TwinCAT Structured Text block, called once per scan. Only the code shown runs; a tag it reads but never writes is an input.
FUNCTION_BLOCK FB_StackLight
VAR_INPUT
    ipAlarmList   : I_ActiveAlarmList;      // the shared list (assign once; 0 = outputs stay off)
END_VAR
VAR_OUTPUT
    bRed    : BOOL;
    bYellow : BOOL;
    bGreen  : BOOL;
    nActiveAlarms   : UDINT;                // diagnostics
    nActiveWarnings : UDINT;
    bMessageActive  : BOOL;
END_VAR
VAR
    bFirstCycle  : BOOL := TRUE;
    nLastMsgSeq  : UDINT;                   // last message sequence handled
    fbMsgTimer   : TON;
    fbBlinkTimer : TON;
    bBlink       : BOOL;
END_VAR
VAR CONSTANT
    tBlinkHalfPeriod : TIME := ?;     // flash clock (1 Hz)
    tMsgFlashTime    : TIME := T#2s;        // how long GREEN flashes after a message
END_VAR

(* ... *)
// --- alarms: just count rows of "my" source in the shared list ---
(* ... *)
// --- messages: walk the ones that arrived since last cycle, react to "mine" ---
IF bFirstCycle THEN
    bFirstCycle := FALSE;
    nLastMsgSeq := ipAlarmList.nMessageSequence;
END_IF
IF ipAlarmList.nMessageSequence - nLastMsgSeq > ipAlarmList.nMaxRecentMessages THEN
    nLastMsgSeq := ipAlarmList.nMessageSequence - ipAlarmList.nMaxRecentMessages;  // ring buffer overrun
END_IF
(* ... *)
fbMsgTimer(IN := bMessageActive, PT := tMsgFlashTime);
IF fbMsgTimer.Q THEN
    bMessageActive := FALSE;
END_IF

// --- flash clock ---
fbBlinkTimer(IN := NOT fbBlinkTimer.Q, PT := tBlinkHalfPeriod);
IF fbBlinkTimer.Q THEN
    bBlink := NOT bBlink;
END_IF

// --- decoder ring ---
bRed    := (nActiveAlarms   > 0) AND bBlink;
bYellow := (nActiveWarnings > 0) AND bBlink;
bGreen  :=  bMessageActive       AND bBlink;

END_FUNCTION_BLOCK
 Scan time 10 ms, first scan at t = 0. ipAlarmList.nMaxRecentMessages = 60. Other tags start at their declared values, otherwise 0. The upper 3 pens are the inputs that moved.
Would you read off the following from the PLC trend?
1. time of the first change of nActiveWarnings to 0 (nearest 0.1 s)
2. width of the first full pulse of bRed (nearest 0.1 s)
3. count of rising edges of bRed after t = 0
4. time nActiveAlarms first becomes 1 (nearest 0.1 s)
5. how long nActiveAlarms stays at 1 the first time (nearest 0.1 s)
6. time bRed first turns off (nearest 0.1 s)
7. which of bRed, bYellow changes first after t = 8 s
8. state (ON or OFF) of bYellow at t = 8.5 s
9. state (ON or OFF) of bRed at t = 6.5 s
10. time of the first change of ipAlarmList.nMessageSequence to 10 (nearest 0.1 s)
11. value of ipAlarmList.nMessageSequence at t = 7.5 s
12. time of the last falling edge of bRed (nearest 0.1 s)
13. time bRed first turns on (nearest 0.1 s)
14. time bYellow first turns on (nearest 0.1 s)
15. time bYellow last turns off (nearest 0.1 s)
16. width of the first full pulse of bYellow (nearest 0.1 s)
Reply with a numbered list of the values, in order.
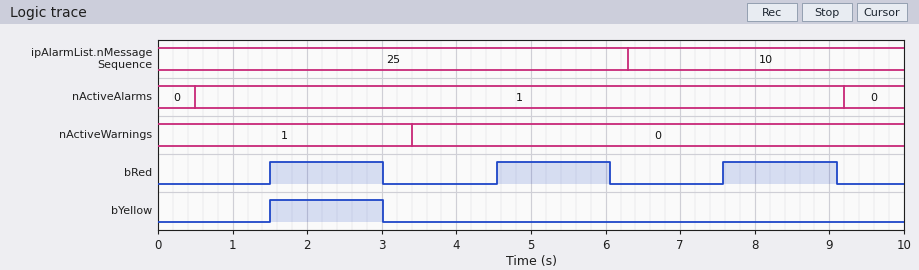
1. 3.4 s
2. 1.5 s
3. 3
4. 0.5 s
5. 8.7 s
6. 3.0 s
7. bRed
8. OFF
9. OFF
10. 6.3 s
11. 10
12. 9.1 s
13. 1.5 s
14. 1.5 s
15. 3.0 s
16. 1.5 s
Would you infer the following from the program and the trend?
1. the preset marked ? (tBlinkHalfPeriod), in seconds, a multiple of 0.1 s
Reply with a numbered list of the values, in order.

1. 1.5 s
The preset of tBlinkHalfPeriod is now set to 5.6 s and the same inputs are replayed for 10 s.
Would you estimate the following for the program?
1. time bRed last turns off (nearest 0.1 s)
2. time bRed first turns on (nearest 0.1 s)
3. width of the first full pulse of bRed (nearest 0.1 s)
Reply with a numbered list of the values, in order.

1. 9.2 s
2. 5.6 s
3. 3.6 s
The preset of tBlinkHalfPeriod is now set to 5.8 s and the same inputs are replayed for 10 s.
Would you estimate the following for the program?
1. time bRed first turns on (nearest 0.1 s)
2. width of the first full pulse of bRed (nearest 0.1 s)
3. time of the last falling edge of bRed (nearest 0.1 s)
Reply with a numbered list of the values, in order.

1. 5.8 s
2. 3.4 s
3. 9.2 s
